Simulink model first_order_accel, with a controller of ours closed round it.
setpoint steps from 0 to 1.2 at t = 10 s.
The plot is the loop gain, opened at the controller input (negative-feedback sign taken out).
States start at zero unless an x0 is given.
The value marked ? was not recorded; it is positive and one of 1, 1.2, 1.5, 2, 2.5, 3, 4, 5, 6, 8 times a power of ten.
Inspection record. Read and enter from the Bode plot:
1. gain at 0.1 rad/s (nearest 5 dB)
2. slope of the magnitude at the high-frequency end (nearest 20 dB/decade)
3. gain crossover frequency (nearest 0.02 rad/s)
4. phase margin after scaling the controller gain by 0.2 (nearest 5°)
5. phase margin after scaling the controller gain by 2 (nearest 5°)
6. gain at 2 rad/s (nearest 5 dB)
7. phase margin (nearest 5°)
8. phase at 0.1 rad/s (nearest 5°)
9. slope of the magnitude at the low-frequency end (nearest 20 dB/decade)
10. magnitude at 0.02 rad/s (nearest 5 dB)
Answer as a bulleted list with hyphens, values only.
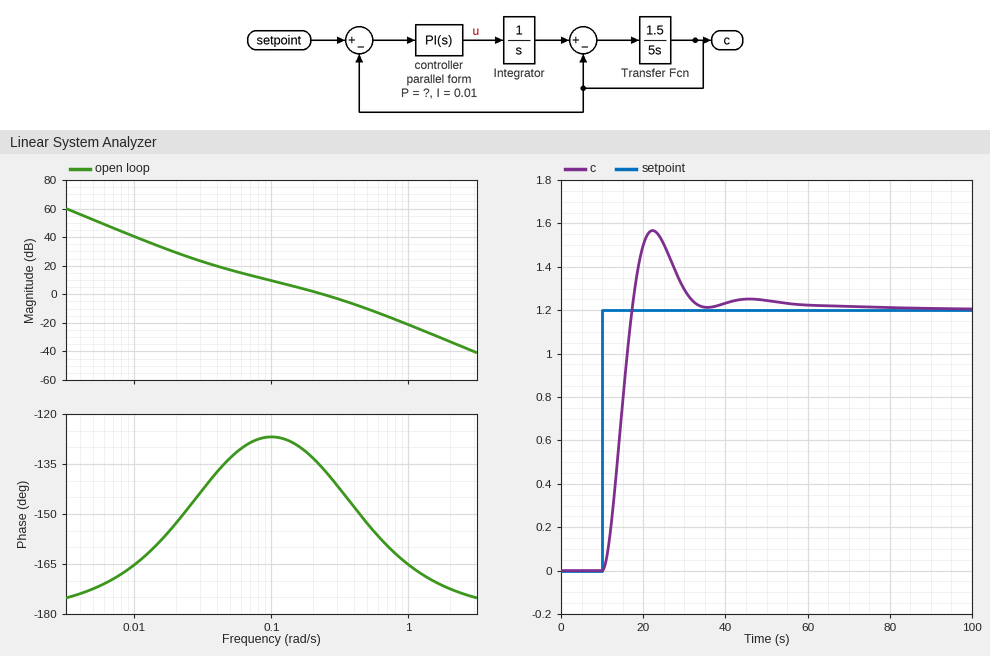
- 10 dB
- -40 dB/decade
- 0.24 rad/s
- 50°
- 35°
- -35 dB
- 45°
- -125°
- -40 dB/decade
- 30 dB
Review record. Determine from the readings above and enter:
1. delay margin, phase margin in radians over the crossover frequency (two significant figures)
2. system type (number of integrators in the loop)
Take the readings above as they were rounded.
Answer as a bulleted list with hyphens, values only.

- 3.3 s
- 2
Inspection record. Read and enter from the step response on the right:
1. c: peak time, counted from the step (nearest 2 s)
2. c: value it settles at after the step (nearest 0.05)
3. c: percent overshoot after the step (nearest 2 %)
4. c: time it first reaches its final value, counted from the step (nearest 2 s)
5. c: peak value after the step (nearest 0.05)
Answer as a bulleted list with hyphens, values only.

- 12 s
- 1.20
- 30 %
- 8 s
- 1.55
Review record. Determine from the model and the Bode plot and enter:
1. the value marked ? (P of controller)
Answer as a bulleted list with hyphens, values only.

- 0.3
